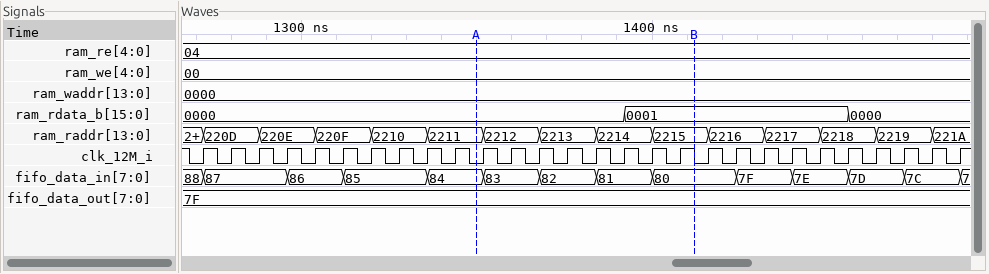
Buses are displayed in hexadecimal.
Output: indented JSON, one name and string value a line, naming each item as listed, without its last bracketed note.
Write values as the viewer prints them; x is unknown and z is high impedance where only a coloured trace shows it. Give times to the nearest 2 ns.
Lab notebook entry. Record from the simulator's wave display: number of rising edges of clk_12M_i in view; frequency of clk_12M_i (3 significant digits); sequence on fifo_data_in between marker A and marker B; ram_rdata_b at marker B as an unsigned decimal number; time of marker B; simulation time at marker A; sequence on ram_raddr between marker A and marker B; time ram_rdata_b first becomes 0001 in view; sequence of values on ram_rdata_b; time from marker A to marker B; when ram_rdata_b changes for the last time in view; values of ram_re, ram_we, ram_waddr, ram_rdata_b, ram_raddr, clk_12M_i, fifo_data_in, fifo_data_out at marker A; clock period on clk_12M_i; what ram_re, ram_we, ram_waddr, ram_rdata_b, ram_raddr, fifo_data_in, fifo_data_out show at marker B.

{
  "number of rising edges of clk_12M_i in view": "28",
  "frequency of clk_12M_i": "125 MHz",
  "sequence on fifo_data_in between marker A and marker B": "84, 83, 82, 81, 80",
  "ram_rdata_b at marker B as an unsigned decimal number": "1",
  "time of marker B": "1412 ns",
  "simulation time at marker A": "1350 ns",
  "sequence on ram_raddr between marker A and marker B": "2211, 2212, 2213, 2214, 2215",
  "time ram_rdata_b first becomes 0001 in view": "1392 ns",
  "sequence of values on ram_rdata_b": "0000, 0001, 0000",
  "time from marker A to marker B": "62 ns",
  "when ram_rdata_b changes for the last time in view": "1456 ns",
  "values of ram_re, ram_we, ram_waddr, ram_rdata_b, ram_raddr, clk_12M_i, fifo_data_in, fifo_data_out at marker A": "ram_re=04, ram_we=00, ram_waddr=0000, ram_rdata_b=0000, ram_raddr=2211, clk_12M_i=0, fifo_data_in=84, fifo_data_out=7F",
  "clock period on clk_12M_i": "8 ns",
  "what ram_re, ram_we, ram_waddr, ram_rdata_b, ram_raddr, fifo_data_in, fifo_data_out show at marker B": "ram_re=04, ram_we=00, ram_waddr=0000, ram_rdata_b=0001, ram_raddr=2215, fifo_data_in=80, fifo_data_out=7F"
}
